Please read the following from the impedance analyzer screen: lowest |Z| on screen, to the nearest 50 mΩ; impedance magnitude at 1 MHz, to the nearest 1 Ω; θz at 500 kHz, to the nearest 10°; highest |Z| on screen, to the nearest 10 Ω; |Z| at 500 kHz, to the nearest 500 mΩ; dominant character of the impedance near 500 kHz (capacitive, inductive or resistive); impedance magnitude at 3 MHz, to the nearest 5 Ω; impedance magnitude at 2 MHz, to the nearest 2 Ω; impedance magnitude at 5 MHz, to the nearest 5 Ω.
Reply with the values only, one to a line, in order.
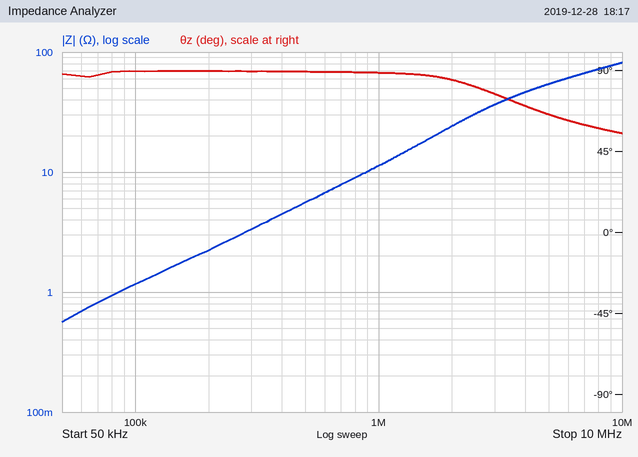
550 mΩ
11 Ω
90°
80 Ω
5.5 Ω
inductive
35 Ω
24 Ω
55 Ω
